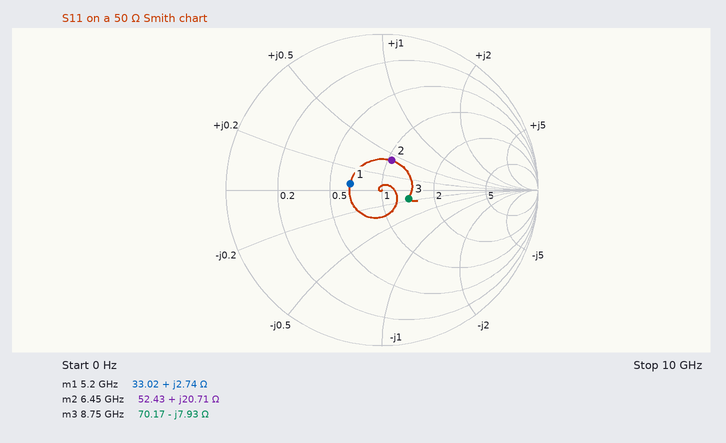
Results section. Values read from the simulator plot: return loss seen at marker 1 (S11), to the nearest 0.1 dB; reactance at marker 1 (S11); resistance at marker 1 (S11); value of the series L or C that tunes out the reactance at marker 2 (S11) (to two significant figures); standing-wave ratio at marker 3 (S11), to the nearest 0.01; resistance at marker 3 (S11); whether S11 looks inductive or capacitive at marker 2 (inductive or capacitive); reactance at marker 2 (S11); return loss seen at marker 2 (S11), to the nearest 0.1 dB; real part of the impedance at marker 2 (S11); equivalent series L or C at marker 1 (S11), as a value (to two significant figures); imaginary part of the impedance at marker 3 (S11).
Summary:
13.7 dB
+2.74 Ω
33.02 Ω
1.2 pF
1.44
70.17 Ω
inductive
+20.71 Ω
14.0 dB
52.43 Ω
84 pH
-7.93 Ω
